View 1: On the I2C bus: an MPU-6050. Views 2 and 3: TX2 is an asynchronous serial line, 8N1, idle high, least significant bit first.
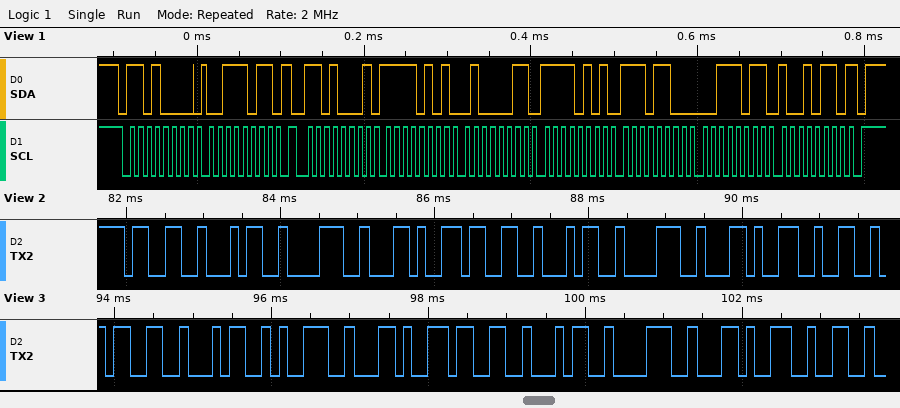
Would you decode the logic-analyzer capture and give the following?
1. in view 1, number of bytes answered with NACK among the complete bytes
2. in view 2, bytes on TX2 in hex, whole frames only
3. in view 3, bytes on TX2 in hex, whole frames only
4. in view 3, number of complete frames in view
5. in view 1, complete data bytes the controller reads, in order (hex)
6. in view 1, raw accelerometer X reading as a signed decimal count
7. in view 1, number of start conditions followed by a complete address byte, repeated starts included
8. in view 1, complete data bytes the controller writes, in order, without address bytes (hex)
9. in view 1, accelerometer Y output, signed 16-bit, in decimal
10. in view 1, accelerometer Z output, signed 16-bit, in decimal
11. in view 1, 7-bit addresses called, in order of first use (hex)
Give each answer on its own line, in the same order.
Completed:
1
33 34 38 2C 33 34 38 2C 32
0x33 0x34 0x39 0x2C 0x33 0x34 0x38 0x2C 0x32
9
F5 43 F5 EC 3B 96
-2749
2
3B
-2580
15254
0x68
